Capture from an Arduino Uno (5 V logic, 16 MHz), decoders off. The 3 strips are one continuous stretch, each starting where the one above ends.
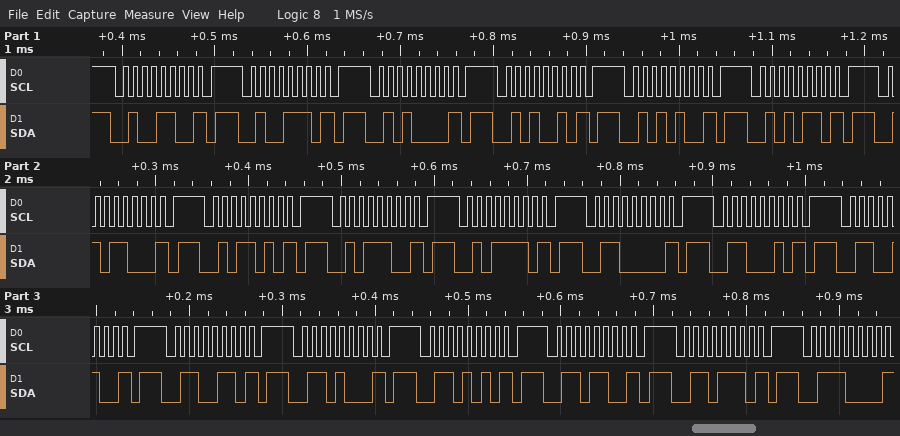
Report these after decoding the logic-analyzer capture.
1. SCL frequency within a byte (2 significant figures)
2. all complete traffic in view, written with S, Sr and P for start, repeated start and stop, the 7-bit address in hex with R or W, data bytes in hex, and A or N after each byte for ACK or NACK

100 kHz
S 26W N P S 27W N P S 28W N P S 29W N P S 2AW N P S 2BW N P S 2CW N P S 2DW N P S 2EW N P S 2FW N P S 30W N P S 31W N P S 32W N P S 33W N P S 34W N P S 35W N P S 36W N P S 37W N P S 38W N
